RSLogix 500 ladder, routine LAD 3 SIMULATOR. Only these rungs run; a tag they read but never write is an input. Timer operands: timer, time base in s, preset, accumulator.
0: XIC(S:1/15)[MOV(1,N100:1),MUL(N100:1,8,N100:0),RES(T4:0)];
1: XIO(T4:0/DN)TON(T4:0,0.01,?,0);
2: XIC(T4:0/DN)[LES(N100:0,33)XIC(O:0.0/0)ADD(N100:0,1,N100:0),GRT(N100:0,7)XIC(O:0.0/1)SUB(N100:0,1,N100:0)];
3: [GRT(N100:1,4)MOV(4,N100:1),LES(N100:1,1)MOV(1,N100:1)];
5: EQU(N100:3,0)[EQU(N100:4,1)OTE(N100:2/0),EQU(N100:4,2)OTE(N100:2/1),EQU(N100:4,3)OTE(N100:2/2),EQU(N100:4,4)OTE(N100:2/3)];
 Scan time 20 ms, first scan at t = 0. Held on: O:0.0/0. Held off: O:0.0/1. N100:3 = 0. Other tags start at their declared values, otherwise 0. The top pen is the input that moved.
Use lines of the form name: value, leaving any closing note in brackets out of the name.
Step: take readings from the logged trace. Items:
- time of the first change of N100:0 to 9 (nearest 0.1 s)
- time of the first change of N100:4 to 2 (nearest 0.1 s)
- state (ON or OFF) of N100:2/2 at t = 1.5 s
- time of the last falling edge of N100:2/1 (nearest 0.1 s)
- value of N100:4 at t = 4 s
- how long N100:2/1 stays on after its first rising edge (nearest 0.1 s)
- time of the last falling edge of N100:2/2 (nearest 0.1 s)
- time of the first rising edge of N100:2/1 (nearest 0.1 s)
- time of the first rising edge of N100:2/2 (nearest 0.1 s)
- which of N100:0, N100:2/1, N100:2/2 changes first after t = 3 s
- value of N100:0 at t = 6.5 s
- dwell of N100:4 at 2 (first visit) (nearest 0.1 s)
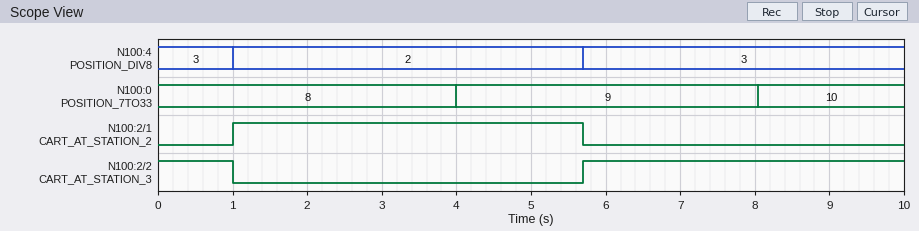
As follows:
time of the first change of N100:0 to 9: 4.0 s
time of the first change of N100:4 to 2: 1.0 s
state (ON or OFF) of N100:2/2 at t = 1.5 s: OFF
time of the last falling edge of N100:2/1: 5.7 s
value of N100:4 at t = 4 s: 2
how long N100:2/1 stays on after its first rising edge: 4.7 s
time of the last falling edge of N100:2/2: 1.0 s
time of the first rising edge of N100:2/1: 1.0 s
time of the first rising edge of N100:2/2: 5.7 s
which of N100:0, N100:2/1, N100:2/2 changes first after t = 3 s: N100:0
value of N100:0 at t = 6.5 s: 9
dwell of N100:4 at 2 (first visit): 4.7 s
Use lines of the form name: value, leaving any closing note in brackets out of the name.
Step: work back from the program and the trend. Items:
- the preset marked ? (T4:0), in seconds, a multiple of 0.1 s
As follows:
the preset marked ? (T4:0), in seconds, a multiple of 0.1 s: 4.0 s
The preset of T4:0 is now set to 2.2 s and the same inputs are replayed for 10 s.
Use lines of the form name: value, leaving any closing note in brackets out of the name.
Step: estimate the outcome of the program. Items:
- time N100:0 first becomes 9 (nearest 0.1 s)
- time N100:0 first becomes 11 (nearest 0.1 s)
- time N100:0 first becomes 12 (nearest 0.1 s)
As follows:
time N100:0 first becomes 9: 2.2 s
time N100:0 first becomes 11: 6.7 s
time N100:0 first becomes 12: 8.9 s
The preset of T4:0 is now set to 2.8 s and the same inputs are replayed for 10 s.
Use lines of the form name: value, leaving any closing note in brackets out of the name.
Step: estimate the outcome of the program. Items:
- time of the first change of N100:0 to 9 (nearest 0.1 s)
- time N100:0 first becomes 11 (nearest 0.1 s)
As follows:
time of the first change of N100:0 to 9: 2.8 s
time N100:0 first becomes 11: 8.5 s
